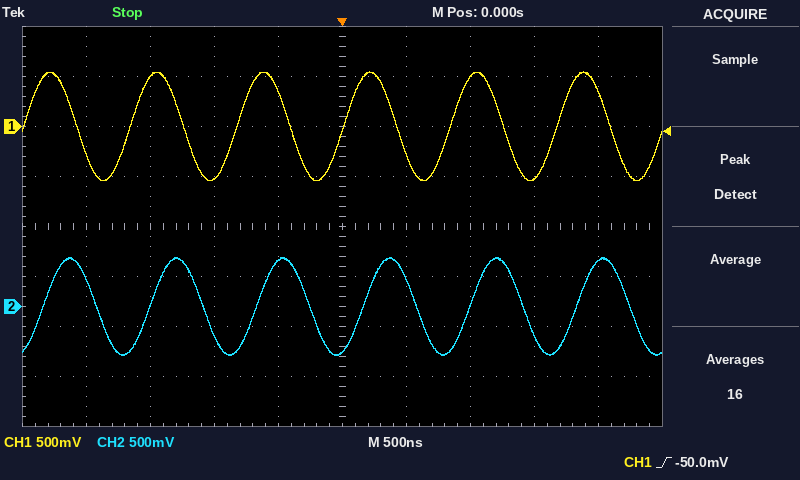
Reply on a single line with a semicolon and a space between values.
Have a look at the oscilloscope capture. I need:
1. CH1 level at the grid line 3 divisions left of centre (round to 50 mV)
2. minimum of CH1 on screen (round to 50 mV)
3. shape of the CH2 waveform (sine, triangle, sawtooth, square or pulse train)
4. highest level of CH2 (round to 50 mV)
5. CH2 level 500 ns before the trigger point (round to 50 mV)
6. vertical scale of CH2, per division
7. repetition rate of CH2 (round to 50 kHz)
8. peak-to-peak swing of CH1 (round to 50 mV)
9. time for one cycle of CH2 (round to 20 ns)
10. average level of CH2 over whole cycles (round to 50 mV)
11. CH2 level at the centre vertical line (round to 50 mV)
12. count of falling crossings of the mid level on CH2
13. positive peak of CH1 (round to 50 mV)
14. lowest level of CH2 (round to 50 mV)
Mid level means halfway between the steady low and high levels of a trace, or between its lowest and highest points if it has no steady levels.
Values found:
500 mV; -550 mV; sine; 500 mV; 450 mV; 500 mV; 1.20 MHz; 1.10 V; 840 ns; 0 mV; -450 mV; 6; 550 mV; -500 mV
